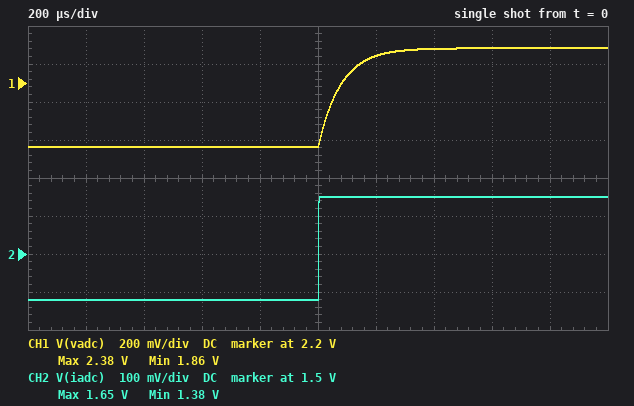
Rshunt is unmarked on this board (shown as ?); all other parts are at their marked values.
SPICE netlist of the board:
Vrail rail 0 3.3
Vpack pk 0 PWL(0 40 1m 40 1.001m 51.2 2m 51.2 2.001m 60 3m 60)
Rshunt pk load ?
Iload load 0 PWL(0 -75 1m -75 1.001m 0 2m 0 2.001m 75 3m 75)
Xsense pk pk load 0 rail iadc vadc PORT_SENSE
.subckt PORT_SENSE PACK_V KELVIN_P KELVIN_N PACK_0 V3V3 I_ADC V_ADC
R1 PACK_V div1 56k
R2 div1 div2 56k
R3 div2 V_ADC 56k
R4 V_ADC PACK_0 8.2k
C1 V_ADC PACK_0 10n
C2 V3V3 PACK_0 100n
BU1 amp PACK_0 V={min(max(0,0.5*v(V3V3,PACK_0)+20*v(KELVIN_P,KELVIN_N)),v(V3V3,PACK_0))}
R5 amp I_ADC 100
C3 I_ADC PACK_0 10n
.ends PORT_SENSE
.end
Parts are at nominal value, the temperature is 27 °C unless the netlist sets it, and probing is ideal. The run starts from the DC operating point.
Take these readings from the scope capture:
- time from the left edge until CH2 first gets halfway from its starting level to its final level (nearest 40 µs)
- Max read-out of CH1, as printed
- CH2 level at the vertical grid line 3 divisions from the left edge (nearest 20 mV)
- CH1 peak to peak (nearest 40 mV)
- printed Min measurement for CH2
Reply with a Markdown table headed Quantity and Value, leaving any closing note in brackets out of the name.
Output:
| Quantity | Value |
|---|---|
| time from the left edge until CH2 first gets halfway from its starting level to its final level | 1.00 ms |
| Max read-out of CH1, as printed | 2.38 V |
| CH2 level at the vertical grid line 3 divisions from the left edge | 1.38 V |
| CH1 peak to peak | 520 mV |
| printed Min measurement for CH2 | 1.38 V |
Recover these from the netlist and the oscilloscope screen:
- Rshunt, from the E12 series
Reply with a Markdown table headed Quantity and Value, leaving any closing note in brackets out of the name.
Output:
| Quantity | Value |
|---|---|
| Rshunt, from the E12 series | 180 µΩ |
